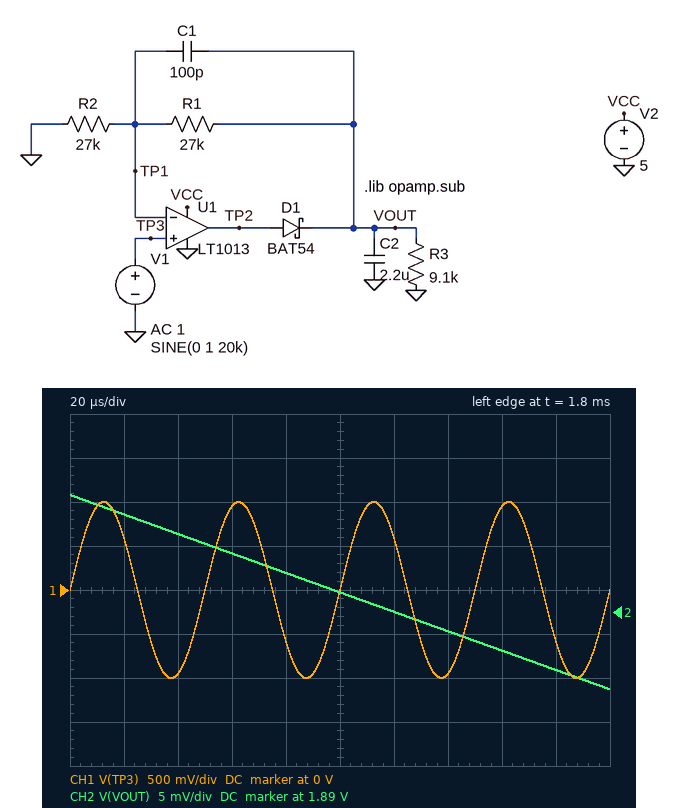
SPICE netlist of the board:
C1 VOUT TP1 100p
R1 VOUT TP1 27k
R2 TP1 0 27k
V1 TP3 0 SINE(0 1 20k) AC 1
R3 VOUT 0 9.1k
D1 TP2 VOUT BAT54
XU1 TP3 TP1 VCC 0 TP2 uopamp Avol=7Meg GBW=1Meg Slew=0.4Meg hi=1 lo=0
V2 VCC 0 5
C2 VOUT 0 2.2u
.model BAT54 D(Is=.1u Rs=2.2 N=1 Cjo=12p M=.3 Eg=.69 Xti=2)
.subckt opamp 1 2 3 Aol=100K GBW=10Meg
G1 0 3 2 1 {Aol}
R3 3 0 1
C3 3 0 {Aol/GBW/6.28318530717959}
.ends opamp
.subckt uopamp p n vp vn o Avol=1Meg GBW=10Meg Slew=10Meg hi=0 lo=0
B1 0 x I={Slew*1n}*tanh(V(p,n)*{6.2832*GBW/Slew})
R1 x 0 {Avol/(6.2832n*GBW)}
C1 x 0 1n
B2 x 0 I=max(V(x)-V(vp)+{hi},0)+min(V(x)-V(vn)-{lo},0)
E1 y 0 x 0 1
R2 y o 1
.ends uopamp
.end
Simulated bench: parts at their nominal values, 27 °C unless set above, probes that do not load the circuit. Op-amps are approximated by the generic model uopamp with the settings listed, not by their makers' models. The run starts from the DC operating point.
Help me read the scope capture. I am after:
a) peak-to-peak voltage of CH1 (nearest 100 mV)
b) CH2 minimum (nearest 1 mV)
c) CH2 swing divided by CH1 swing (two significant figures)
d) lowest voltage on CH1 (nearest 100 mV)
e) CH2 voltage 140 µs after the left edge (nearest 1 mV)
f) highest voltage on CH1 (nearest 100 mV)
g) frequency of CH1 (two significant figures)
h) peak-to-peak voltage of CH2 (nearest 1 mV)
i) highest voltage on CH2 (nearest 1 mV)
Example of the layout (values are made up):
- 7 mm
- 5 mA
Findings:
- 2.0 V
- 1.881 V
- 0.011
- -1.0 V
- 1.888 V
- 1.0 V
- 20 kHz
- 22 mV
- 1.903 V
